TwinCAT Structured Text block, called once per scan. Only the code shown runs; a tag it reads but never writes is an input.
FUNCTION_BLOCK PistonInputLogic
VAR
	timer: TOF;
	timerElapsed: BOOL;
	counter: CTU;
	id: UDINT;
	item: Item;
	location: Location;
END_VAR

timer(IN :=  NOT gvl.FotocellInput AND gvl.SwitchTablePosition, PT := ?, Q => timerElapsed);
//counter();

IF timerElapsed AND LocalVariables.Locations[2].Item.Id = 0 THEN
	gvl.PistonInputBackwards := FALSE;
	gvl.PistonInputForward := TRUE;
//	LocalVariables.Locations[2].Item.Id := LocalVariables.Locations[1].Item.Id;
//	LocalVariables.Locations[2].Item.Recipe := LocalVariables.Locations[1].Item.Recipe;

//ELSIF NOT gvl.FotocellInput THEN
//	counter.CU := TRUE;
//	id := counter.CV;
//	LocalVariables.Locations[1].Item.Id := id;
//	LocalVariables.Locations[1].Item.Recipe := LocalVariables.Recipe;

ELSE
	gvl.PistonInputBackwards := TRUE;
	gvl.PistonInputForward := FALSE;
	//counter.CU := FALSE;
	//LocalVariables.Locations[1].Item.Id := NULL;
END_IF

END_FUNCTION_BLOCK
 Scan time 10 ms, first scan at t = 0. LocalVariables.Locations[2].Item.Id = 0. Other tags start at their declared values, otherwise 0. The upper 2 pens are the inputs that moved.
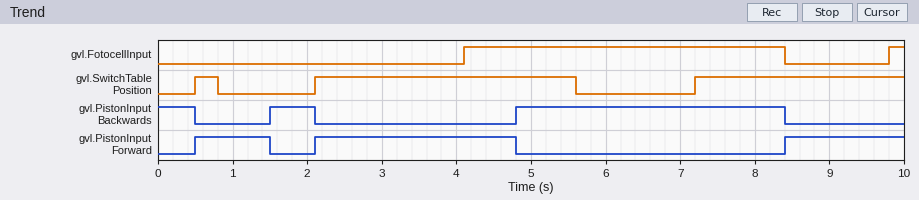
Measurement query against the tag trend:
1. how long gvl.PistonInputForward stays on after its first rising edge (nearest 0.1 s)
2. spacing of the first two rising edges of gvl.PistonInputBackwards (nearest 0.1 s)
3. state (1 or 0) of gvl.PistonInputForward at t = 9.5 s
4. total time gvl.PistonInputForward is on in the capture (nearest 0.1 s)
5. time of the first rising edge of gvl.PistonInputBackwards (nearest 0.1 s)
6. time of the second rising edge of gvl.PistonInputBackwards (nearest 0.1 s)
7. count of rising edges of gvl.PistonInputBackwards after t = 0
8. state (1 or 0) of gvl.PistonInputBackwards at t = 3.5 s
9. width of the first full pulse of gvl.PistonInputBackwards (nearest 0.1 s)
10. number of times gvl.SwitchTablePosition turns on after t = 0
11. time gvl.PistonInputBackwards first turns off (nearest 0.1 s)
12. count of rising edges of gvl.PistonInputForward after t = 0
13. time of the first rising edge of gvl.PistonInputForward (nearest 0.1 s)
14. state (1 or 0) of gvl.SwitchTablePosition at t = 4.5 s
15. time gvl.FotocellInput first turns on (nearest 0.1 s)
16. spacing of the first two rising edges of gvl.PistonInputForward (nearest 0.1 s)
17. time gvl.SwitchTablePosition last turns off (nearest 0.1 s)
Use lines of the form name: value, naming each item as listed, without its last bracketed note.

how long gvl.PistonInputForward stays on after its first rising edge: 1.0 s
spacing of the first two rising edges of gvl.PistonInputBackwards: 3.3 s
state (1 or 0) of gvl.PistonInputForward at t = 9.5 s: 1
total time gvl.PistonInputForward is on in the capture: 5.3 s
time of the first rising edge of gvl.PistonInputBackwards: 1.5 s
time of the second rising edge of gvl.PistonInputBackwards: 4.8 s
count of rising edges of gvl.PistonInputBackwards after t = 0: 2
state (1 or 0) of gvl.PistonInputBackwards at t = 3.5 s: 0
width of the first full pulse of gvl.PistonInputBackwards: 0.6 s
number of times gvl.SwitchTablePosition turns on after t = 0: 3
time gvl.PistonInputBackwards first turns off: 0.5 s
count of rising edges of gvl.PistonInputForward after t = 0: 3
time of the first rising edge of gvl.PistonInputForward: 0.5 s
state (1 or 0) of gvl.SwitchTablePosition at t = 4.5 s: 1
time gvl.FotocellInput first turns on: 4.1 s
spacing of the first two rising edges of gvl.PistonInputForward: 1.6 s
time gvl.SwitchTablePosition last turns off: 5.6 s
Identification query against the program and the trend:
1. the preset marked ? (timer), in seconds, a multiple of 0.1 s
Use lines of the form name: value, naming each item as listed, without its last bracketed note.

the preset marked ? (timer), in seconds, a multiple of 0.1 s: 0.7 s
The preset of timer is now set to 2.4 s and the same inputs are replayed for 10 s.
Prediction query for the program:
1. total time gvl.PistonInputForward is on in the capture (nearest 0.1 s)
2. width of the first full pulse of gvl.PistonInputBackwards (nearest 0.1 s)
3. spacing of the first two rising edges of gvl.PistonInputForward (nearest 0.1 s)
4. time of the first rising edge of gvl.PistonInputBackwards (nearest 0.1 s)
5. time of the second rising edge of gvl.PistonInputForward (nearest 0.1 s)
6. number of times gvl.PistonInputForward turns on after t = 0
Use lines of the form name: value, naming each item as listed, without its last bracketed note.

total time gvl.PistonInputForward is on in the capture: 7.6 s
width of the first full pulse of gvl.PistonInputBackwards: 1.9 s
spacing of the first two rising edges of gvl.PistonInputForward: 7.9 s
time of the first rising edge of gvl.PistonInputBackwards: 6.5 s
time of the second rising edge of gvl.PistonInputForward: 8.4 s
number of times gvl.PistonInputForward turns on after t = 0: 2
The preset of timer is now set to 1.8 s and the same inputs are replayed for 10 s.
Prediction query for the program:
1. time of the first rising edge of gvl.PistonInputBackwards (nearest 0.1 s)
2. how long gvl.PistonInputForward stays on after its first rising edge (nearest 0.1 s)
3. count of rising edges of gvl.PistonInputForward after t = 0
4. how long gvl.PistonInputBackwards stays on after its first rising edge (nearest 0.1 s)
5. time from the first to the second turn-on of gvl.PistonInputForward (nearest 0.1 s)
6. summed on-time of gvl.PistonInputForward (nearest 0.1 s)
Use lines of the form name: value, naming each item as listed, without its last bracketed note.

time of the first rising edge of gvl.PistonInputBackwards: 5.9 s
how long gvl.PistonInputForward stays on after its first rising edge: 5.4 s
count of rising edges of gvl.PistonInputForward after t = 0: 2
how long gvl.PistonInputBackwards stays on after its first rising edge: 2.5 s
time from the first to the second turn-on of gvl.PistonInputForward: 7.9 s
summed on-time of gvl.PistonInputForward: 7.0 s
